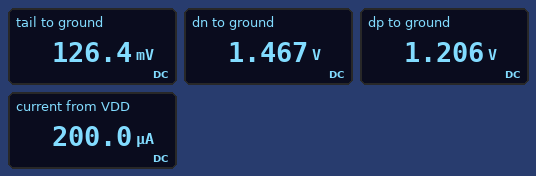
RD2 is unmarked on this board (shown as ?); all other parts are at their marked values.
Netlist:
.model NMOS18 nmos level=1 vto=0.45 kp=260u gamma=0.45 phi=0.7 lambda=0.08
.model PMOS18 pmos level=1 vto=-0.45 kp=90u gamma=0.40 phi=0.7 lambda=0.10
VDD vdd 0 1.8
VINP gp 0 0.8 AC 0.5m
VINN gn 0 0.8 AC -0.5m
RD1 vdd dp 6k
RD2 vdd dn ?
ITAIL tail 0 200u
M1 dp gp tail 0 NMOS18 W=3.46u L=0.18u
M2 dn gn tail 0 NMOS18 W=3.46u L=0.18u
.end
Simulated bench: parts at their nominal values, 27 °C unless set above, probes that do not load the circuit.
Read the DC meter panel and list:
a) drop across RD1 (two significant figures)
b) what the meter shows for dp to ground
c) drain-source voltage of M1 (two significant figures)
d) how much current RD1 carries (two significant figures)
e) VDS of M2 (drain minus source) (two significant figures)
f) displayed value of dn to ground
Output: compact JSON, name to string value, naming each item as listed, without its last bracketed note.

{"drop across RD1": "590 mV", "what the meter shows for dp to ground": "1.206 V", "drain-source voltage of M1": "1.1 V", "how much current RD1 carries": "99 µA", "VDS of M2 (drain minus source)": "1.3 V", "displayed value of dn to ground": "1.467 V"}
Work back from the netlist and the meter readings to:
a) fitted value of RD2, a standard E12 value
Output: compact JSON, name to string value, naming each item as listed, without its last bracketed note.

{"fitted value of RD2, a standard E12 value": "3.3 kΩ"}
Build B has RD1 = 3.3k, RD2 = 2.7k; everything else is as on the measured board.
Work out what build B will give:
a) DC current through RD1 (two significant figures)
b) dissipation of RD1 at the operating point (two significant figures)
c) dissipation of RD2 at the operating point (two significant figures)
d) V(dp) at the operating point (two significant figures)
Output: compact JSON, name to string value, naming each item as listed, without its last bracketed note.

{"DC current through RD1": "100 µA", "dissipation of RD1 at the operating point": "33 µW", "dissipation of RD2 at the operating point": "27 µW", "V(dp) at the operating point": "1.5 V"}
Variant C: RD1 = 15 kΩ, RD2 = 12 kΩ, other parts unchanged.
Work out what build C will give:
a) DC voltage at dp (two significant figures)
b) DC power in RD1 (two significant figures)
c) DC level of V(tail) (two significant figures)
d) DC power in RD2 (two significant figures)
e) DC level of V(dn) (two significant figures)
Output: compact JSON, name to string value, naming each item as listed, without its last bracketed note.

{"DC voltage at dp": "320 mV", "DC power in RD1": "150 µW", "DC level of V(tail)": "120 mV", "DC power in RD2": "120 µW", "DC level of V(dn)": "590 mV"}
